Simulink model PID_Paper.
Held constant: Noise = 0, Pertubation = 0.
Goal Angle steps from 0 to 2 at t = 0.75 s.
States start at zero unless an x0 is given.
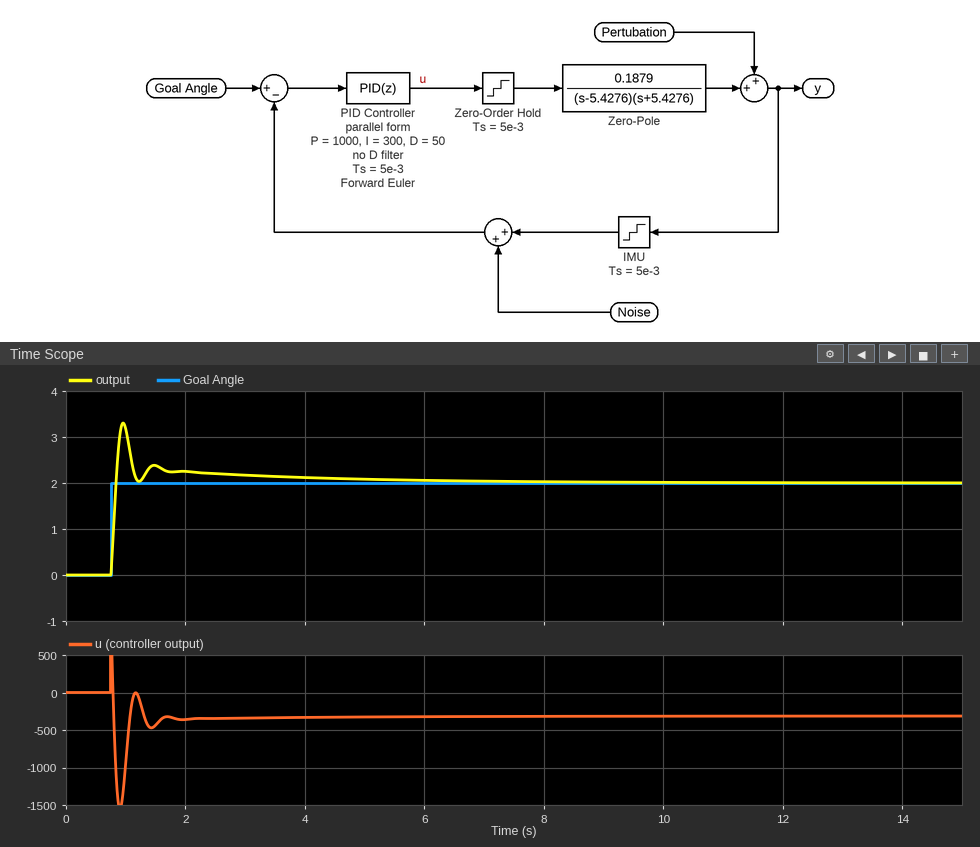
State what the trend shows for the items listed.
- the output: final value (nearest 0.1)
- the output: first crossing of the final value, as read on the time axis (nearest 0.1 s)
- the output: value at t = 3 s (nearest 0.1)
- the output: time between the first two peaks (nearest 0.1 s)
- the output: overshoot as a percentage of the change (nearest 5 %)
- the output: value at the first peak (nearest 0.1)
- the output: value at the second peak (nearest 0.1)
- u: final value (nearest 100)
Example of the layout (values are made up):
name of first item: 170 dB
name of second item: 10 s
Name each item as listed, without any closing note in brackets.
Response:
the output: final value: 2.0
the output: first crossing of the final value, as read on the time axis: 0.8 s
the output: value at t = 3 s: 2.2
the output: time between the first two peaks: 0.5 s
the output: overshoot as a percentage of the change: 65 %
the output: value at the first peak: 3.3
the output: value at the second peak: 2.4
u: final value: -300
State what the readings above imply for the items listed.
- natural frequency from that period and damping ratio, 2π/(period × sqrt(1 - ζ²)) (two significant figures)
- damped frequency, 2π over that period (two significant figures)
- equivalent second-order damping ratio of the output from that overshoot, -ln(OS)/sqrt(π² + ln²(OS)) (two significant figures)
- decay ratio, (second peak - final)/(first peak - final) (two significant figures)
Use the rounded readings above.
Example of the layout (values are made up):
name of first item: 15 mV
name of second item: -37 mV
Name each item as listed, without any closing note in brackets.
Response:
natural frequency from that period and damping ratio, 2π/(period × sqrt(1 - ζ²)): 13 rad/s
damped frequency, 2π over that period: 13 rad/s
equivalent second-order damping ratio of the output from that overshoot, -ln(OS)/sqrt(π² + ln²(OS)): 0.14
decay ratio, (second peak - final)/(first peak - final): 0.31
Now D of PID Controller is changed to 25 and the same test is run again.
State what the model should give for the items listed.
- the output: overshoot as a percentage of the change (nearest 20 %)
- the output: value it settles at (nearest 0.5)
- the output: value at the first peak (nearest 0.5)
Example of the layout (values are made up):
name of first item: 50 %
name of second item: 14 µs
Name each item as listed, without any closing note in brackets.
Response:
the output: overshoot as a percentage of the change: 100 %
the output: value it settles at: 2.0
the output: value at the first peak: 4.0
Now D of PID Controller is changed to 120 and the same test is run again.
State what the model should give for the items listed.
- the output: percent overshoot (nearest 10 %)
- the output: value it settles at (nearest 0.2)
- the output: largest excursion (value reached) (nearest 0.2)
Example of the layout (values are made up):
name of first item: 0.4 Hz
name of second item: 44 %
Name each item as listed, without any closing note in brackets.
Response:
the output: percent overshoot: 30 %
the output: value it settles at: 2.0
the output: largest excursion (value reached): 2.6
